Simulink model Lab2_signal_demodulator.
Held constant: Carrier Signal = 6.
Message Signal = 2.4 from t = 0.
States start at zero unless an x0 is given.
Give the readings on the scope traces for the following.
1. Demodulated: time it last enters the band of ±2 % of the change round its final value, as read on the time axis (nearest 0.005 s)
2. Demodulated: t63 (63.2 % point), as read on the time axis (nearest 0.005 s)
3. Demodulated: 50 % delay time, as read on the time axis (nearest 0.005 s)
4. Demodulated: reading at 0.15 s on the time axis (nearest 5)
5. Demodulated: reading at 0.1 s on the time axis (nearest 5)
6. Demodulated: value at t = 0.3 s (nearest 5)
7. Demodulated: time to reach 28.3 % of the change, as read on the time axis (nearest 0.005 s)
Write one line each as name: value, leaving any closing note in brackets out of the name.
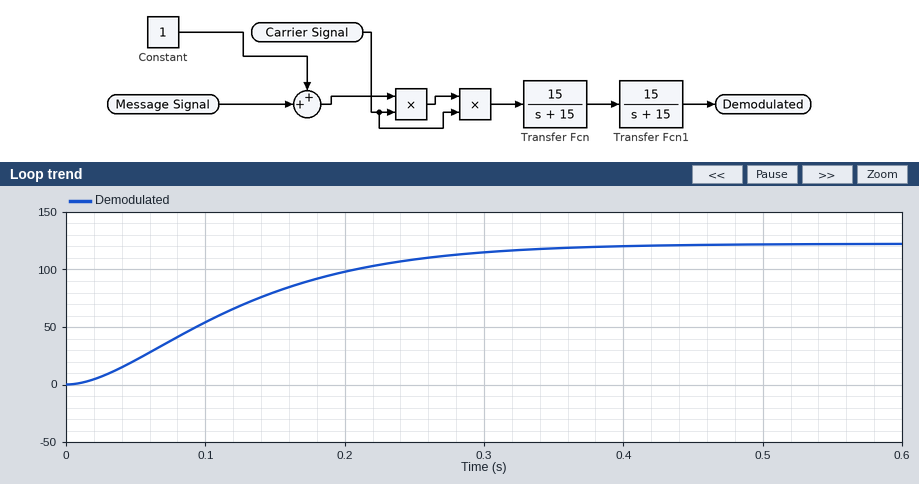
Demodulated: time it last enters the band of ±2 % of the change round its final value, as read on the time axis: 0.390 s
Demodulated: t63 (63.2 % point), as read on the time axis: 0.145 s
Demodulated: 50 % delay time, as read on the time axis: 0.110 s
Demodulated: reading at 0.15 s on the time axis: 80
Demodulated: reading at 0.1 s on the time axis: 55
Demodulated: value at t = 0.3 s: 115
Demodulated: time to reach 28.3 % of the change, as read on the time axis: 0.070 s
